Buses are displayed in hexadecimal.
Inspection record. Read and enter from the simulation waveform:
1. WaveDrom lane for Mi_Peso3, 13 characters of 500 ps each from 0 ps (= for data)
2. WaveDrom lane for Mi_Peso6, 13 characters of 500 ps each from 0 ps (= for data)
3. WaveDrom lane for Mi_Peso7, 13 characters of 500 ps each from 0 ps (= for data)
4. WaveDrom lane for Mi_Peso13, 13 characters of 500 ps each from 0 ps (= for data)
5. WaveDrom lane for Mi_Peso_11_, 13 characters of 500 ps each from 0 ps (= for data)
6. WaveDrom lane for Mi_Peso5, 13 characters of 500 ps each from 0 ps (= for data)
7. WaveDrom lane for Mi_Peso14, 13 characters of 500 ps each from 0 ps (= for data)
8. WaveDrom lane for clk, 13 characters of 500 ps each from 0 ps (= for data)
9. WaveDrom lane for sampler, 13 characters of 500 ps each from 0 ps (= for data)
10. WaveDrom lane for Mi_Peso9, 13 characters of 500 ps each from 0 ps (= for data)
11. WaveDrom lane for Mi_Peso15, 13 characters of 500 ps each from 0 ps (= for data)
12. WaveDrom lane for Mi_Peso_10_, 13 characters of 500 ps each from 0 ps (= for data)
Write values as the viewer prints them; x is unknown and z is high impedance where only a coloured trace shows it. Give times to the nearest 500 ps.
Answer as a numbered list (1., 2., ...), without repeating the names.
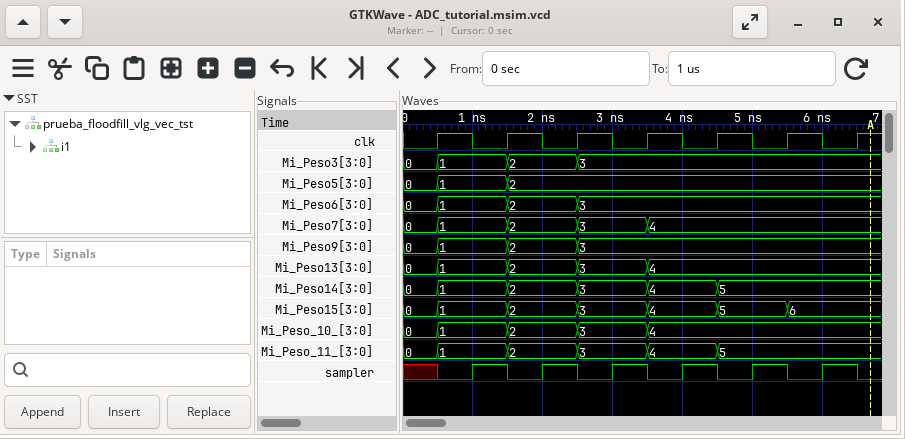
1. {name: 'Mi_Peso3', wave: '==.=.=.......', data: '0 1 2 3'}
2. {name: 'Mi_Peso6', wave: '==.=.=.......', data: '0 1 2 3'}
3. {name: 'Mi_Peso7', wave: '==.=.=.=.....', data: '0 1 2 3 4'}
4. {name: 'Mi_Peso13', wave: '==.=.=.=.....', data: '0 1 2 3 4'}
5. {name: 'Mi_Peso_11_', wave: '==.=.=.=.=...', data: '0 1 2 3 4 5'}
6. {name: 'Mi_Peso5', wave: '==.=.........', data: '0 1 2'}
7. {name: 'Mi_Peso14', wave: '==.=.=.=.=...', data: '0 1 2 3 4 5'}
8. {name: 'clk', wave: '0101010101010'}
9. {name: 'sampler', wave: 'x010101010101'}
10. {name: 'Mi_Peso9', wave: '==.=.=.......', data: '0 1 2 3'}
11. {name: 'Mi_Peso15', wave: '==.=.=.=.=.=.', data: '0 1 2 3 4 5 6'}
12. {name: 'Mi_Peso_10_', wave: '==.=.=.=.....', data: '0 1 2 3 4'}
